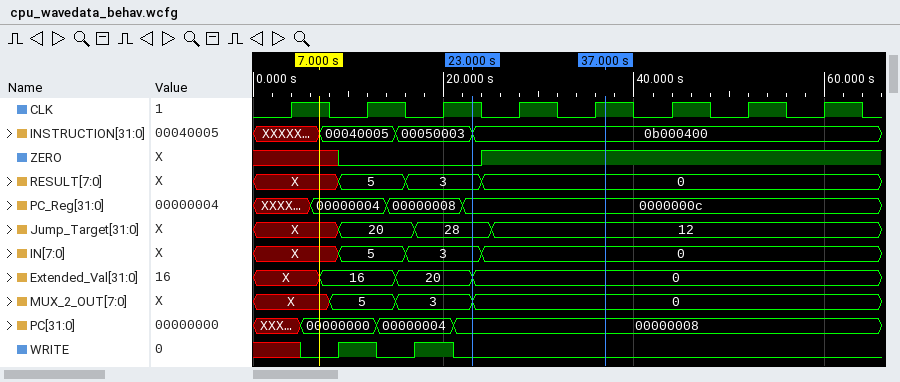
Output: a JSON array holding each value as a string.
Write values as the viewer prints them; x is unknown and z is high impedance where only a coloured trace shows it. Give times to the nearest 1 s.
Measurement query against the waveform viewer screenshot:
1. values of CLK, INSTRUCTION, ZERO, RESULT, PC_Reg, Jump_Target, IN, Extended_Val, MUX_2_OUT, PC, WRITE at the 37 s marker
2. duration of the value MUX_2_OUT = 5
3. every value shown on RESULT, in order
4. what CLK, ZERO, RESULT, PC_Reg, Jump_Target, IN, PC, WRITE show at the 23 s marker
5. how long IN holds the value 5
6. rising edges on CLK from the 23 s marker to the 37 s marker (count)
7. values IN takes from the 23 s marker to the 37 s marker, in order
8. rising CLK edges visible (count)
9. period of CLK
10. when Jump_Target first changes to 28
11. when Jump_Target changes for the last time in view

["CLK=1, INSTRUCTION=0b000400, ZERO=1, RESULT=0, PC_Reg=0000000c, Jump_Target=12, IN=0, Extended_Val=0, MUX_2_OUT=0, PC=00000008, WRITE=0", "7 s", "X, 5, 3, 0", "CLK=1, ZERO=0, RESULT=3, PC_Reg=0000000c, Jump_Target=28, IN=3, PC=00000008, WRITE=0", "7 s", "2", "3, 0", "8", "8 s", "17 s", "25 s"]
